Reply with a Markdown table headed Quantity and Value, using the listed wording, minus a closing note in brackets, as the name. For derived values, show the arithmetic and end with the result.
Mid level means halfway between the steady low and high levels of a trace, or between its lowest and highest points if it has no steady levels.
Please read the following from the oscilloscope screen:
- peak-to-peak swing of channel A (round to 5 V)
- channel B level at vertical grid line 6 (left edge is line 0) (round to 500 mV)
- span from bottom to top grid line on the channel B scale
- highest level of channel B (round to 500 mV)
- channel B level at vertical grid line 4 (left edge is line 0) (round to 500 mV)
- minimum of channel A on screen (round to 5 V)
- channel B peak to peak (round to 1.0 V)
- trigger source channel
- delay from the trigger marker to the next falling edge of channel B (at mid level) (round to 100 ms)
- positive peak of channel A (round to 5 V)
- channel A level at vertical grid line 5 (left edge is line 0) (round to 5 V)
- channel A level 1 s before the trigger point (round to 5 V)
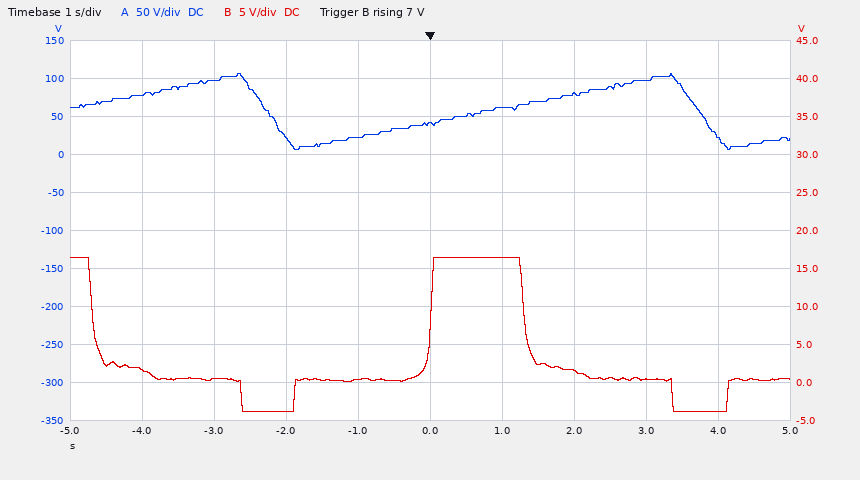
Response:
| Quantity | Value |
|---|---|
| peak-to-peak swing of channel A | 105 V − (5 V) = 100 V |
| channel B level at vertical grid line 6 (left edge is line 0) | 16.5 V |
| span from bottom to top grid line on the channel B scale | 50 V |
| highest level of channel B | 16.5 V |
| channel B level at vertical grid line 4 (left edge is line 0) | 500 mV |
| minimum of channel A on screen | 5 V |
| channel B peak to peak | 20.0 V |
| trigger source channel | channel B |
| delay from the trigger marker to the next falling edge of channel B (at mid level) | 1.3 s |
| positive peak of channel A | 105 V |
| channel A level at vertical grid line 5 (left edge is line 0) | 40 V |
| channel A level 1 s before the trigger point | 20 V |
